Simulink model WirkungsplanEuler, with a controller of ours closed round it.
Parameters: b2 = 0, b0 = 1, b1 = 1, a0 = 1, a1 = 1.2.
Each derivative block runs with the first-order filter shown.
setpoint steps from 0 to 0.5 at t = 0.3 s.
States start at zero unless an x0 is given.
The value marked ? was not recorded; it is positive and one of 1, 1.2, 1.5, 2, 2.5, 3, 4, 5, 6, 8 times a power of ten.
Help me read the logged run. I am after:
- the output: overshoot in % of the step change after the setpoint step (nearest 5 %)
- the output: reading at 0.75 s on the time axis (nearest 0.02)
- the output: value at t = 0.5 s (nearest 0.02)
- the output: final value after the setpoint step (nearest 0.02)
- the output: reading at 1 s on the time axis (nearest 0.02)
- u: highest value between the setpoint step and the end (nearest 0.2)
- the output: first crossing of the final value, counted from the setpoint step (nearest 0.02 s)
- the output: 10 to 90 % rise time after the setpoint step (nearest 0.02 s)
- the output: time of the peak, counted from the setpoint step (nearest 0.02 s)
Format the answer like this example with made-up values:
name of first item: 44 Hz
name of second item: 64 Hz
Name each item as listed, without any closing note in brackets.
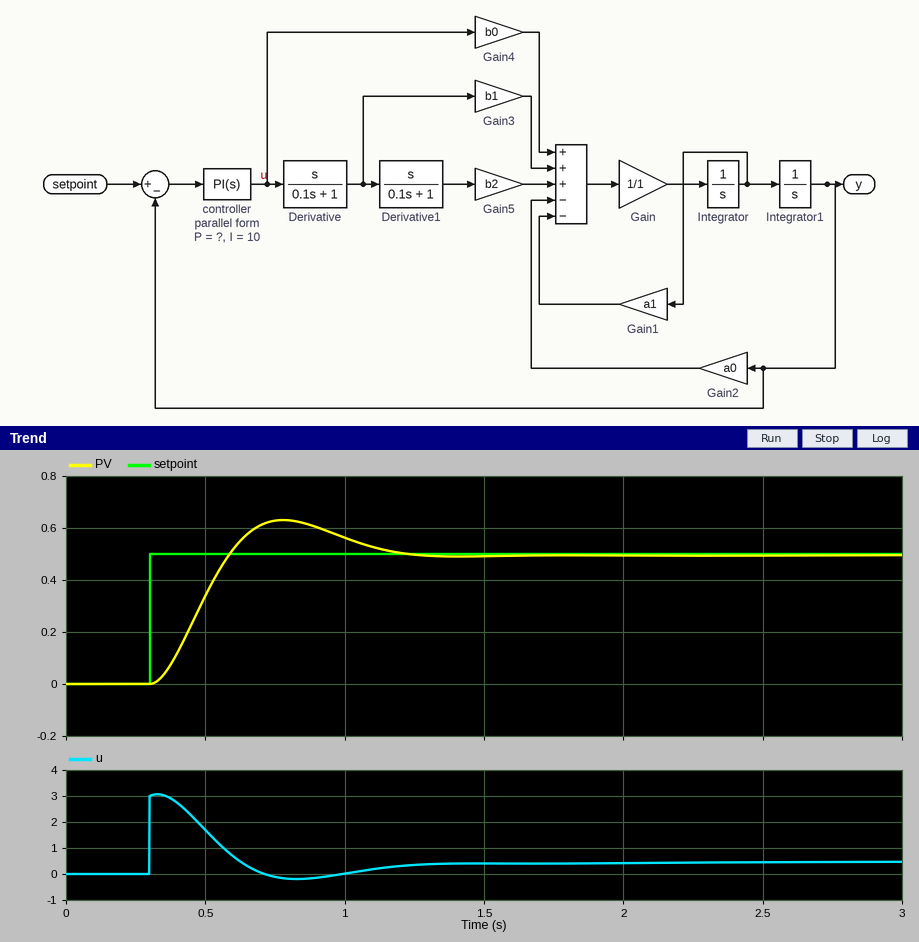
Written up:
the output: overshoot in % of the step change after the setpoint step: 25 %
the output: reading at 0.75 s on the time axis: 0.62
the output: value at t = 0.5 s: 0.34
the output: final value after the setpoint step: 0.50
the output: reading at 1 s on the time axis: 0.56
u: highest value between the setpoint step and the end: 3.0
the output: first crossing of the final value, counted from the setpoint step: 0.28 s
the output: 10 to 90 % rise time after the setpoint step: 0.20 s
the output: time of the peak, counted from the setpoint step: 0.48 s
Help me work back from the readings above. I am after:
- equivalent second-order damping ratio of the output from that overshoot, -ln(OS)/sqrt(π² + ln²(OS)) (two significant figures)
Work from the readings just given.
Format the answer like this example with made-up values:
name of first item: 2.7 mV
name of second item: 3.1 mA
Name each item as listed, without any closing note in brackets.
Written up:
equivalent second-order damping ratio of the output from that overshoot, -ln(OS)/sqrt(π² + ln²(OS)): 0.40
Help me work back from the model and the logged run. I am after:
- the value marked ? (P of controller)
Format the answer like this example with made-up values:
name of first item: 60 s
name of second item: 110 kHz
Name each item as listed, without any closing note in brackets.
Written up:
the value marked ?: 6
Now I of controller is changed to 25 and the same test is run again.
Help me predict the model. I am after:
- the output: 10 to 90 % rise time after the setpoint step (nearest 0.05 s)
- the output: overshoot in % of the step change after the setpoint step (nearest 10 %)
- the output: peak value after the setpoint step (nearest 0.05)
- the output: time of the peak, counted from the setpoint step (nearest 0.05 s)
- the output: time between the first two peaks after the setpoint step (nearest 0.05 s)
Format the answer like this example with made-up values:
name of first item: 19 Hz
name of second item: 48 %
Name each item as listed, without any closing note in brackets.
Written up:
the output: 10 to 90 % rise time after the setpoint step: 0.15 s
the output: overshoot in % of the step change after the setpoint step: 50 %
the output: peak value after the setpoint step: 0.75
the output: time of the peak, counted from the setpoint step: 0.45 s
the output: time between the first two peaks after the setpoint step: 1.00 s
